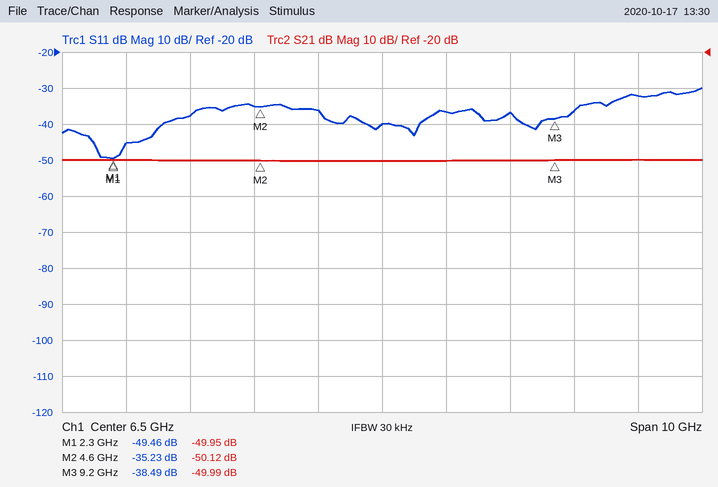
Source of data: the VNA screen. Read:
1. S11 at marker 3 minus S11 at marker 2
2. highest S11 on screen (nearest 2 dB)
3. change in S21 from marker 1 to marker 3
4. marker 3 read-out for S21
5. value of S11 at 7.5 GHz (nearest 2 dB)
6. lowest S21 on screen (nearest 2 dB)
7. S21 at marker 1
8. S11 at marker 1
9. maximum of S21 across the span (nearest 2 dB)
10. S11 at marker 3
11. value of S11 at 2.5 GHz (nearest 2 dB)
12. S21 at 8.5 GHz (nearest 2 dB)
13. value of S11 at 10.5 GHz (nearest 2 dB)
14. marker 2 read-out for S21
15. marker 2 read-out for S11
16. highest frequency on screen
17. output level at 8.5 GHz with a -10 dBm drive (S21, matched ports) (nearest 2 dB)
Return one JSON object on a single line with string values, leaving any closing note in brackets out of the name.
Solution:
{"S11 at marker 3 minus S11 at marker 2": "-3.26 dB", "highest S11 on screen": "-30 dB", "change in S21 from marker 1 to marker 3": "-0.04 dB", "marker 3 read-out for S21": "-49.99 dB", "value of S11 at 7.5 GHz": "-36 dB", "lowest S21 on screen": "-50 dB", "S21 at marker 1": "-49.95 dB", "S11 at marker 1": "-49.46 dB", "maximum of S21 across the span": "-50 dB", "S11 at marker 3": "-38.49 dB", "value of S11 at 2.5 GHz": "-46 dB", "S21 at 8.5 GHz": "-50 dB", "value of S11 at 10.5 GHz": "-32 dB", "marker 2 read-out for S21": "-50.12 dB", "marker 2 read-out for S11": "-35.23 dB", "highest frequency on screen": "11.5 GHz", "output level at 8.5 GHz with a -10 dBm drive (S21, matched ports)": "-60 dBm"}
